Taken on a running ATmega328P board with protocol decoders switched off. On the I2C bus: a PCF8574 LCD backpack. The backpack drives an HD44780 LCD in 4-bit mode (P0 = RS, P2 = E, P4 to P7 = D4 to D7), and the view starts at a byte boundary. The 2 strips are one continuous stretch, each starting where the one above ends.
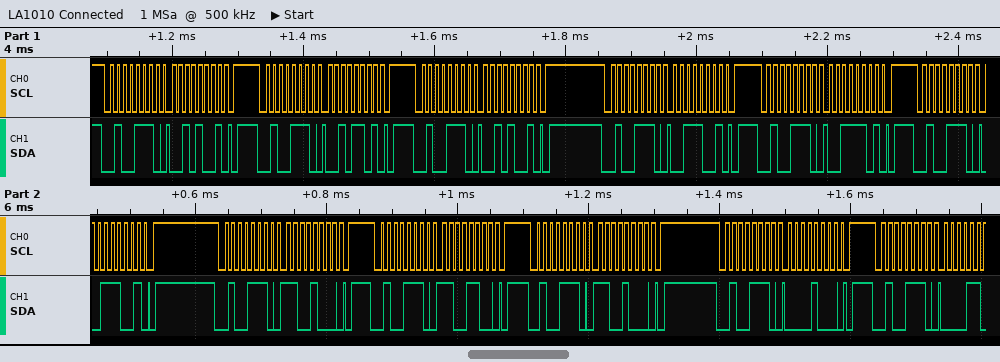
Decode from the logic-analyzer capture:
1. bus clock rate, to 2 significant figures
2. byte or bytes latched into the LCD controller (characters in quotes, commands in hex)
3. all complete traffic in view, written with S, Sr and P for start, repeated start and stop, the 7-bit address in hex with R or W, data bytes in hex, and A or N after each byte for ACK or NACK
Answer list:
100 kHz
'#'
S 27W A 29 A P S 27W A 2D A P S 27W A 29 A P S 27W A 39 A P S 27W A 3D A P S 27W A 39 A P S 27W A C8 A P S 27W A CC A P S 27W A C8 A P S 27W A 08 A P S 27W A
